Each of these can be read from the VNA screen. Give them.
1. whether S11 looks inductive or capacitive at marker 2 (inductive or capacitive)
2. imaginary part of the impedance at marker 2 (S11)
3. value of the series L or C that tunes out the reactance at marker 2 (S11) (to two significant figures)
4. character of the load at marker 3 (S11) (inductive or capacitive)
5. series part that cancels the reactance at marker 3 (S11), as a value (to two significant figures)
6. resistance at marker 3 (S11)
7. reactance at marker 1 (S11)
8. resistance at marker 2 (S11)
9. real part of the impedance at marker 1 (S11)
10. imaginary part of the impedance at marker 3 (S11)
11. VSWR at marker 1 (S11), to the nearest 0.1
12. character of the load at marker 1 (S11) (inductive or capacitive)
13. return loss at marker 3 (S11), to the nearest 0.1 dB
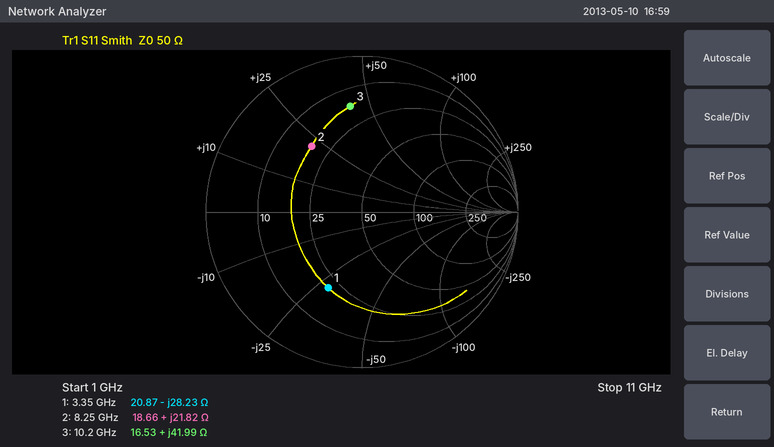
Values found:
inductive
+21.82 Ω
880 fF
inductive
370 fF
16.53 Ω
-28.23 Ω
18.66 Ω
20.87 Ω
+41.99 Ω
3.3
capacitive
3.3 dB
